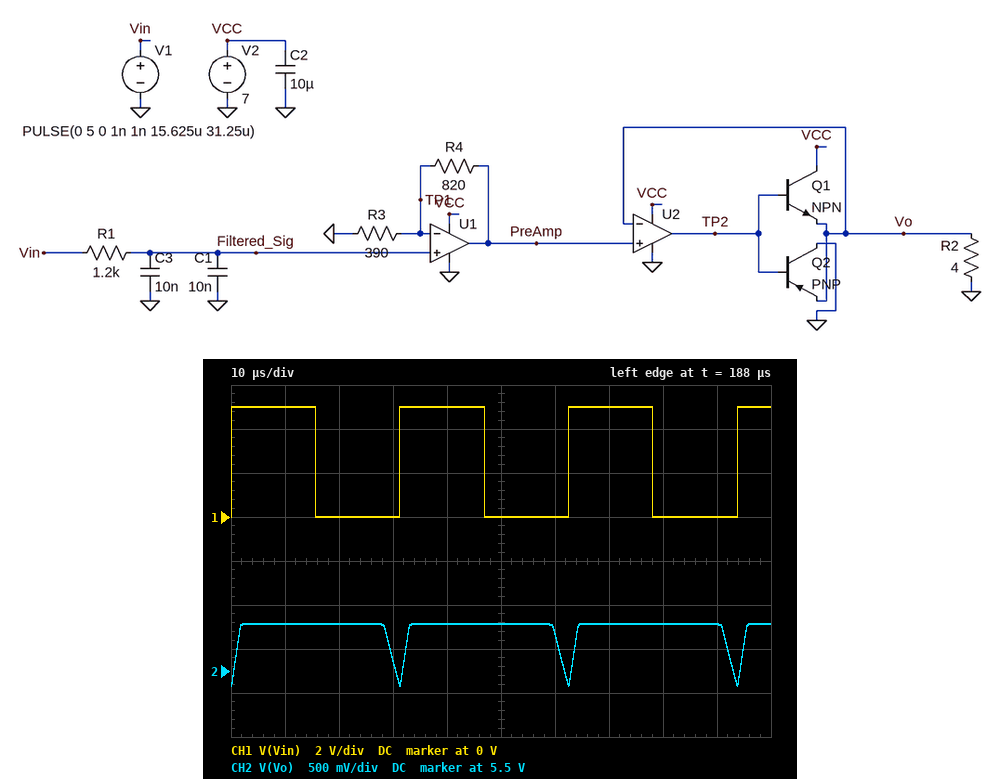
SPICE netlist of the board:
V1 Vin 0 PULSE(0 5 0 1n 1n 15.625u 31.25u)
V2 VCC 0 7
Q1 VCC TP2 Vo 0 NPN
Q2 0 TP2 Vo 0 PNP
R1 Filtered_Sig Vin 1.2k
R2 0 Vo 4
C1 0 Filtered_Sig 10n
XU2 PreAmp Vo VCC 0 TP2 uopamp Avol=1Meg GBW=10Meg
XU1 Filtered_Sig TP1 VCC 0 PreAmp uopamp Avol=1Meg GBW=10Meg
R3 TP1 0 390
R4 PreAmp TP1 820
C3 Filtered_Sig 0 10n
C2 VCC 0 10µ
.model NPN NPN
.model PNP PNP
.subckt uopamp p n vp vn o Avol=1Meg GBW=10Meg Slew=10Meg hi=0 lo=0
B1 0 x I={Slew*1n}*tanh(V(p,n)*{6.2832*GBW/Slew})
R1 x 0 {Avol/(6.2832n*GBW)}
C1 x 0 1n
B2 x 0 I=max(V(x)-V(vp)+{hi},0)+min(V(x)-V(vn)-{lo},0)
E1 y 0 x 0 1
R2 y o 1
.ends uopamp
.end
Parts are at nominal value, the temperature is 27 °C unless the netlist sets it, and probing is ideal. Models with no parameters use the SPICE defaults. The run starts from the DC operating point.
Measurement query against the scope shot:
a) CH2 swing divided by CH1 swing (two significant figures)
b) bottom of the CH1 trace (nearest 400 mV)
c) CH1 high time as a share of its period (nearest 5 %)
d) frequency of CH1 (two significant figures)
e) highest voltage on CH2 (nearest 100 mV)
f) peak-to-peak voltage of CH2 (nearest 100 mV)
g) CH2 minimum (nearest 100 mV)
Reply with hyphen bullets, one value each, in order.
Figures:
- 0.14
- 0 V
- 50 %
- 32 kHz
- 6.0 V
- 700 mV
- 5.3 V
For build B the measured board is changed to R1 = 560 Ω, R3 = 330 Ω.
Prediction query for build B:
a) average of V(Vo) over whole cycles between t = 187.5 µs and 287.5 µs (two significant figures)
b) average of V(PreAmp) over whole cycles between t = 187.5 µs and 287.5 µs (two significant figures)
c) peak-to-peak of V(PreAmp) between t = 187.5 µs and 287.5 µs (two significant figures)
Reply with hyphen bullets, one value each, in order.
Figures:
- 5.7 V
- 6.3 V
- 3.5 V
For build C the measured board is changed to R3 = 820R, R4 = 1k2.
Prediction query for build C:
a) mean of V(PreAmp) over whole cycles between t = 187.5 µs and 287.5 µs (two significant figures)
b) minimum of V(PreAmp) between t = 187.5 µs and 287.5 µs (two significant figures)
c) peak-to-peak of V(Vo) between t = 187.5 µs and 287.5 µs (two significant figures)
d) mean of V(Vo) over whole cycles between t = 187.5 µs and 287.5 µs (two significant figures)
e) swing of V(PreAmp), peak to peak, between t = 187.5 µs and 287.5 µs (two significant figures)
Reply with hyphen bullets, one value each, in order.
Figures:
- 6.0 V
- 4.2 V
- 1.8 V
- 5.6 V
- 2.8 V
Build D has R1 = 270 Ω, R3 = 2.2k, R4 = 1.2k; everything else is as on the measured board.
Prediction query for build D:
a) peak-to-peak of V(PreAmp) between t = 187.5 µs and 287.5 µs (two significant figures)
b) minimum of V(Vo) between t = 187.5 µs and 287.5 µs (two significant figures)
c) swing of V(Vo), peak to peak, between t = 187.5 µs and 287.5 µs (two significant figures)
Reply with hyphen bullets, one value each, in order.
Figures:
- 6.6 V
- 410 mV
- 5.6 V
